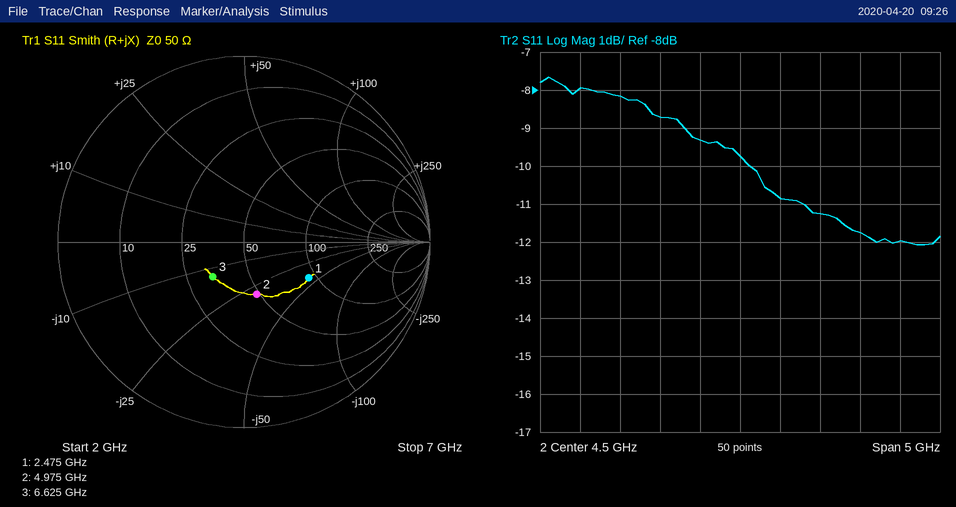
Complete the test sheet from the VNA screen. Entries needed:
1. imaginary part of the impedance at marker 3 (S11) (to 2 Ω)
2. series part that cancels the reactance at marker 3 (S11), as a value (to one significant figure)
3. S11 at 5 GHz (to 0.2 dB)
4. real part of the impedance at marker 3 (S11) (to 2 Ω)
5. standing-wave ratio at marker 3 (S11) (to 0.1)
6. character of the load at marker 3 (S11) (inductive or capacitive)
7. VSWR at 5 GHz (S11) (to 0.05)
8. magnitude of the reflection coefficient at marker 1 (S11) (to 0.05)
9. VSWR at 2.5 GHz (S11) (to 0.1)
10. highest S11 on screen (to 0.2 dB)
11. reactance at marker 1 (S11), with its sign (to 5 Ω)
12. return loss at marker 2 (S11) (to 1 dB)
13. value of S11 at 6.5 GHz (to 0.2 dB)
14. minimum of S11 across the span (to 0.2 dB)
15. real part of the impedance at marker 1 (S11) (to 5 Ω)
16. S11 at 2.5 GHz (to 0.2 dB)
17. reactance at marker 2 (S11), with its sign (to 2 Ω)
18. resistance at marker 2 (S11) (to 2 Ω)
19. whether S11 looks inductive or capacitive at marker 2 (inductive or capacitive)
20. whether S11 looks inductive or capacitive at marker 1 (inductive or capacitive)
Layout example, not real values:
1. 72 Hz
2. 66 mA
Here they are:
1. -14 Ω
2. 300 pH
3. -10.8 dB
4. 34 Ω
5. 1.7
6. capacitive
7. 1.80
8. 0.40
9. 2.3
10. -7.6 dB
11. -40 Ω
12. 11 dB
13. -12.0 dB
14. -12.0 dB
15. 90 Ω
16. -8.0 dB
17. -30 Ω
18. 48 Ω
19. capacitive
20. capacitive
